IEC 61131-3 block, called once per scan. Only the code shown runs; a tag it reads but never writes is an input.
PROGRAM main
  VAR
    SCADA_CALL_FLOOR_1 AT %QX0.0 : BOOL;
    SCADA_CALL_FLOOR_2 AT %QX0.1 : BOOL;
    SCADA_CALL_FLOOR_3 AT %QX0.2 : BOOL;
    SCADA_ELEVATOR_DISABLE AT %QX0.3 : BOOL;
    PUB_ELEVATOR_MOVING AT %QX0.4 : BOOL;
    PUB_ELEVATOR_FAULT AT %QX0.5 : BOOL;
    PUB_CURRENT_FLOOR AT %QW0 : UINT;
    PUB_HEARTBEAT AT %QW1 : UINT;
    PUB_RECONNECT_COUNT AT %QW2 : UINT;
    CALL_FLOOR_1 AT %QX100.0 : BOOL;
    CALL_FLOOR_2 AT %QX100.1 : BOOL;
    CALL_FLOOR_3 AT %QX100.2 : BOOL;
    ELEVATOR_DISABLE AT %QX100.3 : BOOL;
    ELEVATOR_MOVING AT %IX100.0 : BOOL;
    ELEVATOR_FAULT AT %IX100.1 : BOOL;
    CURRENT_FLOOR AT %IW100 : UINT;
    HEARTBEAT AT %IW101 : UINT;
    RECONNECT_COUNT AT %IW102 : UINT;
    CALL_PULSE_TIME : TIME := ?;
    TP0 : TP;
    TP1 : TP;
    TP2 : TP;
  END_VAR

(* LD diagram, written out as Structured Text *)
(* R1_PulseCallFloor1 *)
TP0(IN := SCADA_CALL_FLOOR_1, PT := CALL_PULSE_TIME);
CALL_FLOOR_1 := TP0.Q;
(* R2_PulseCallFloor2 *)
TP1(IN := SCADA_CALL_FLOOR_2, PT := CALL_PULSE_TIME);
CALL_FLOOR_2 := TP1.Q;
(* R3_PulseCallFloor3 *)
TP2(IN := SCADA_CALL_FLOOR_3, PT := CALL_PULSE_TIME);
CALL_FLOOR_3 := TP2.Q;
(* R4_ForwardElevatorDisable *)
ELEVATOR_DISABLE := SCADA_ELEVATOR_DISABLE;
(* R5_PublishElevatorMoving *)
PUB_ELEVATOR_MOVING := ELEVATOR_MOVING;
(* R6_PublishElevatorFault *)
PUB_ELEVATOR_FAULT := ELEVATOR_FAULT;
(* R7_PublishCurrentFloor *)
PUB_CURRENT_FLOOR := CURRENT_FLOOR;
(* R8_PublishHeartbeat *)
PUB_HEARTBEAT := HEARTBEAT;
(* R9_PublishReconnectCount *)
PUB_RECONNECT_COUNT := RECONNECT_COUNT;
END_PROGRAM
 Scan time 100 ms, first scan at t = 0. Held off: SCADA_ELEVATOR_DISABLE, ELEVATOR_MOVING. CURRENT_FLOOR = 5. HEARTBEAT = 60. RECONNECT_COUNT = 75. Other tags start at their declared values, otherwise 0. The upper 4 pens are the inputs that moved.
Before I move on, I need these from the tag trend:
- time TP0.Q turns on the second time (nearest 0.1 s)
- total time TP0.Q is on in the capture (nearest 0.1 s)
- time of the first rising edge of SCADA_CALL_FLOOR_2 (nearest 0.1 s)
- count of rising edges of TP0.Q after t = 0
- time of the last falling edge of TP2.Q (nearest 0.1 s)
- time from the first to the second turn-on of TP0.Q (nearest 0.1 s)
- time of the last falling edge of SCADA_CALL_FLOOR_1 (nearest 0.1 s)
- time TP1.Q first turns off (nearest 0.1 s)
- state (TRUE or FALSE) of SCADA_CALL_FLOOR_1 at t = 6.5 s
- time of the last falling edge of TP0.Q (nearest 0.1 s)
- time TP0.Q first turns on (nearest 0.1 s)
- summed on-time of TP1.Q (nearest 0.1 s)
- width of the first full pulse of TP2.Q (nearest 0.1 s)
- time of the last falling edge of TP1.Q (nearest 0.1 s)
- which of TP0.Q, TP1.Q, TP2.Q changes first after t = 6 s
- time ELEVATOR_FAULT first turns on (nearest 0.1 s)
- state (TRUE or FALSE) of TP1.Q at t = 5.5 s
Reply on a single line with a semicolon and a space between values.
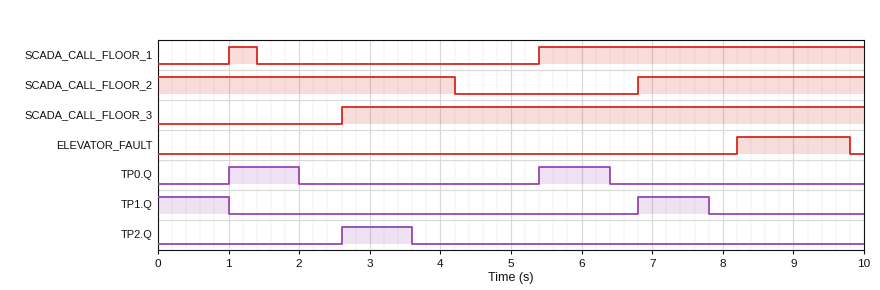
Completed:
5.4 s; 2.0 s; 6.8 s; 2; 3.6 s; 4.4 s; 1.4 s; 1.0 s; TRUE; 6.4 s; 1.0 s; 2.0 s; 1.0 s; 7.8 s; TP0.Q; 8.2 s; FALSE
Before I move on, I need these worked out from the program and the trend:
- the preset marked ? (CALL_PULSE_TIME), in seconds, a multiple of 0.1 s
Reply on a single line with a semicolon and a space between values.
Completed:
1.0 s
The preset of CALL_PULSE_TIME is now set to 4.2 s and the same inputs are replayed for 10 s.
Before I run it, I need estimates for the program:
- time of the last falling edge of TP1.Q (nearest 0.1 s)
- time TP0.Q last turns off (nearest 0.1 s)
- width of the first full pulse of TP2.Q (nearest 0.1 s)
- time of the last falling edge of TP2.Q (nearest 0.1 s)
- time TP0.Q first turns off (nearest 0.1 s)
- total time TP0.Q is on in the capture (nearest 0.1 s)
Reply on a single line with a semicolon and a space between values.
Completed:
4.2 s; 9.6 s; 4.2 s; 6.8 s; 5.2 s; 8.4 s
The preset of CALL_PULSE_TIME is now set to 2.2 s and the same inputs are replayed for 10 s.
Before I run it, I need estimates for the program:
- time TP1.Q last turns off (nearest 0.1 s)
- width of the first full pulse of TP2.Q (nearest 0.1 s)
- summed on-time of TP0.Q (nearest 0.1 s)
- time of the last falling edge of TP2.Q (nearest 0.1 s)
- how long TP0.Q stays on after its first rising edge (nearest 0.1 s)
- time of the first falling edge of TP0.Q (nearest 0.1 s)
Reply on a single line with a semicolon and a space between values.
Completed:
9.0 s; 2.2 s; 4.4 s; 4.8 s; 2.2 s; 3.2 s
